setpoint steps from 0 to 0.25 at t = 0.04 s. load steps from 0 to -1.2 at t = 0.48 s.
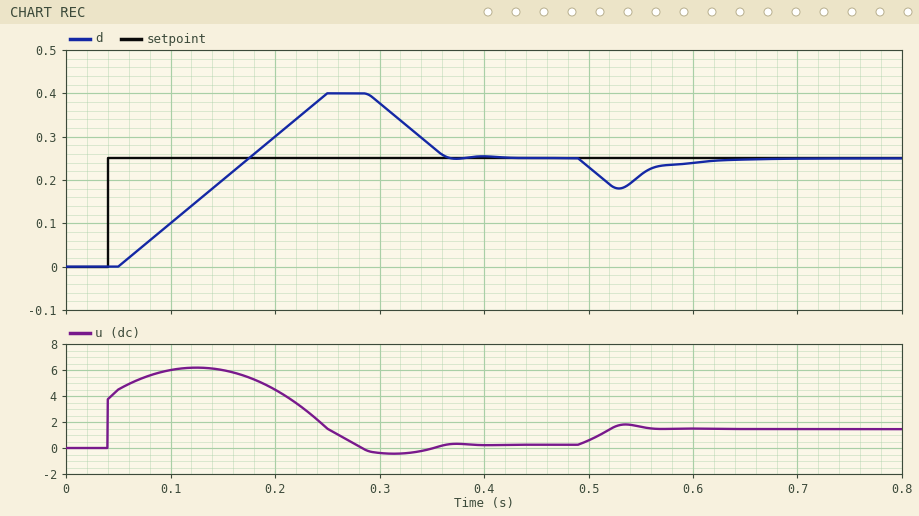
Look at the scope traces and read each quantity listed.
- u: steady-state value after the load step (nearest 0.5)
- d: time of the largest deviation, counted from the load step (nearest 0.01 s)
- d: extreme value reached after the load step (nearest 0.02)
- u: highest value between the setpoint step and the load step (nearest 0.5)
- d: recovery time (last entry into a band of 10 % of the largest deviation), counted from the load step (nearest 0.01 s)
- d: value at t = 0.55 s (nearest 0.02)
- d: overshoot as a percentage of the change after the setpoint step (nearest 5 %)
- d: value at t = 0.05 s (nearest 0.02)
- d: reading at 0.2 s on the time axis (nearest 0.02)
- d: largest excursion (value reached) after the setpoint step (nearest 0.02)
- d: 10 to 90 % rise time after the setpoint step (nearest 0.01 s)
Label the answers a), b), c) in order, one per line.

a) 1.5
b) 0.05 s
c) 0.18
d) 6.0
e) 0.13 s
f) 0.22
g) 60 %
h) 0.00
i) 0.30
j) 0.40
k) 0.10 s
